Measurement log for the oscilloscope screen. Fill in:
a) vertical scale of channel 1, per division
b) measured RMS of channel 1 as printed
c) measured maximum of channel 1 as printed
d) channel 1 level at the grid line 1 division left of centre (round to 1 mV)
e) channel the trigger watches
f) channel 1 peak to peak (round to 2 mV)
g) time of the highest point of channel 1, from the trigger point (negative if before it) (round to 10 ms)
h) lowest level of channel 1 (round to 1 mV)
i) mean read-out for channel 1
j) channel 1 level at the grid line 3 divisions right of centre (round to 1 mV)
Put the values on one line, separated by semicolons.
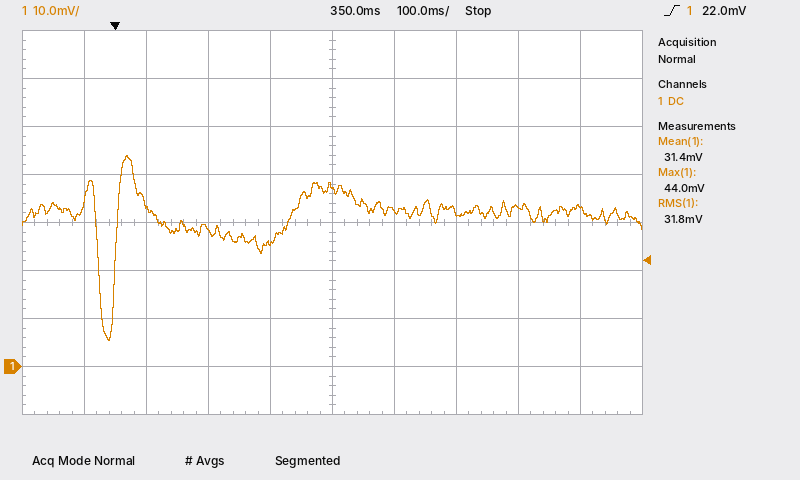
10 mV; 31.8 mV; 44.0 mV; 26 mV; channel 1; 38 mV; +20 ms; 5 mV; 31.4 mV; 33 mV
